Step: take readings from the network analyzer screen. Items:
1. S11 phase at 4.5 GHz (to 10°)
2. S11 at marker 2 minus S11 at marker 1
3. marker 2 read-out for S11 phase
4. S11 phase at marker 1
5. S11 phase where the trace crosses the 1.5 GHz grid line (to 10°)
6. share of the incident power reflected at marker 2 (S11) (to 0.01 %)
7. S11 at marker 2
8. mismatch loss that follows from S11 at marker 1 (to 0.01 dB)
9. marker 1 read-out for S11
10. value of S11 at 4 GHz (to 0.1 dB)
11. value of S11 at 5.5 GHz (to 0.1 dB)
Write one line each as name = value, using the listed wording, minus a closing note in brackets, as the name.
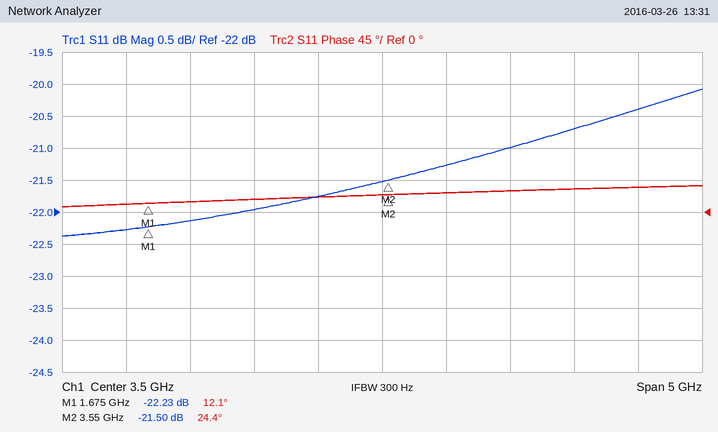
S11 phase at 4.5 GHz = 30°
S11 at marker 2 minus S11 at marker 1 = 0.73 dB
marker 2 read-out for S11 phase = 24.4°
S11 phase at marker 1 = 12.1°
S11 phase where the trace crosses the 1.5 GHz grid line = 10°
share of the incident power reflected at marker 2 (S11) = 0.71 %
S11 at marker 2 = -21.50 dB
mismatch loss that follows from S11 at marker 1 = 0.03 dB
marker 1 read-out for S11 = -22.23 dB
value of S11 at 4 GHz = -21.3 dB
value of S11 at 5.5 GHz = -20.4 dB
